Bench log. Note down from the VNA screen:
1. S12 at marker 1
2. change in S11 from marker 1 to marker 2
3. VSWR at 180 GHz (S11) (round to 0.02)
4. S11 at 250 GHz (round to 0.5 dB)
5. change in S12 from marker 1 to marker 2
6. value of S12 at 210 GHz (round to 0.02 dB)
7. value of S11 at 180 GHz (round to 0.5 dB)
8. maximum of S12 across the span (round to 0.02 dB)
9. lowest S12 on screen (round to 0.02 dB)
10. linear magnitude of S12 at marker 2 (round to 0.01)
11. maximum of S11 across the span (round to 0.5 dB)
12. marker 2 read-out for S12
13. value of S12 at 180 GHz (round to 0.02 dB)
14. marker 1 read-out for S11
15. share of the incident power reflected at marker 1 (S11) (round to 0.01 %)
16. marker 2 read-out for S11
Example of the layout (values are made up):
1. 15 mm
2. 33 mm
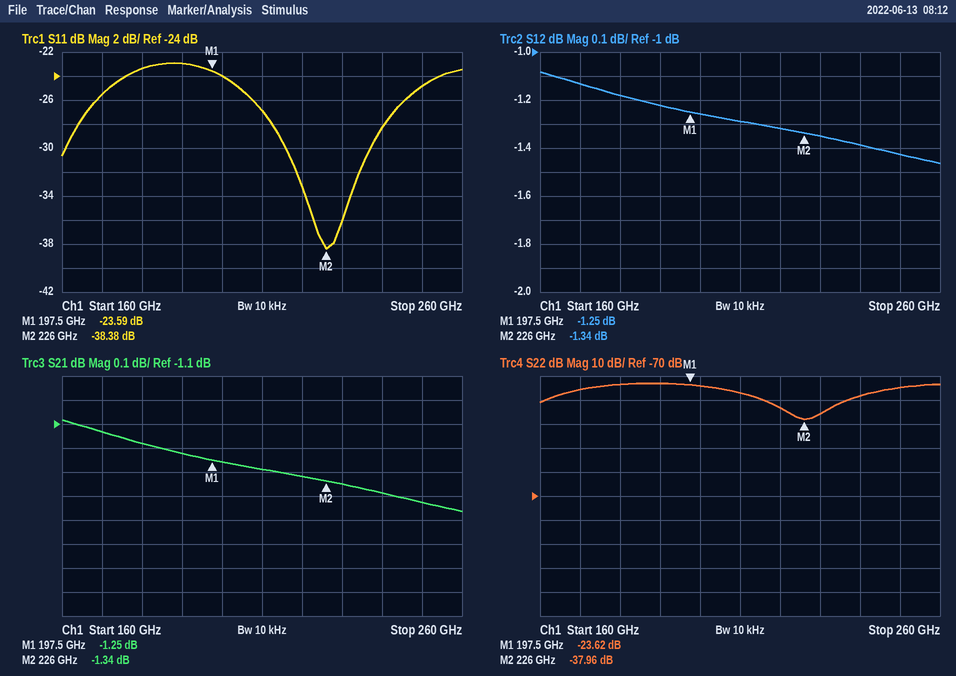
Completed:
1. -1.25 dB
2. -14.79 dB
3. 1.14
4. -25.0 dB
5. -0.09 dB
6. -1.28 dB
7. -23.5 dB
8. -1.08 dB
9. -1.46 dB
10. 0.86
11. -23.0 dB
12. -1.34 dB
13. -1.18 dB
14. -23.59 dB
15. 0.44 %
16. -38.38 dB
